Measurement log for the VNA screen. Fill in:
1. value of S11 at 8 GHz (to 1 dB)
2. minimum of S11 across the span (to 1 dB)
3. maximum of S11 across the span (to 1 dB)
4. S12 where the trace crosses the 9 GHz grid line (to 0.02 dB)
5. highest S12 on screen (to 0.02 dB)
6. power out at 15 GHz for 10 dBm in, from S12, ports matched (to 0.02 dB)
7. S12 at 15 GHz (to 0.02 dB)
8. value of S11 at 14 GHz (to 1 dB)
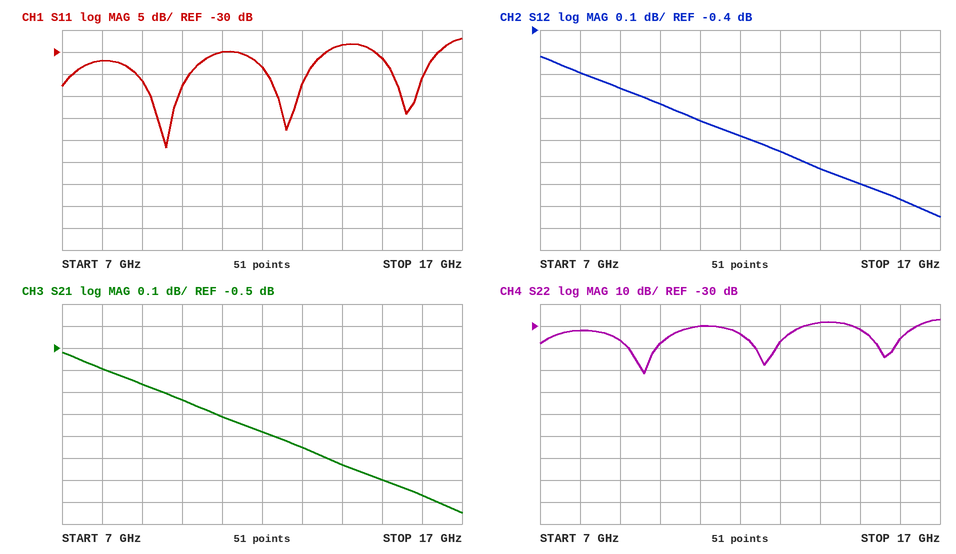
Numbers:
-32 dB
-52 dB
-27 dB
-0.66 dB
-0.52 dB
8.90 dBm
-1.10 dB
-28 dB
